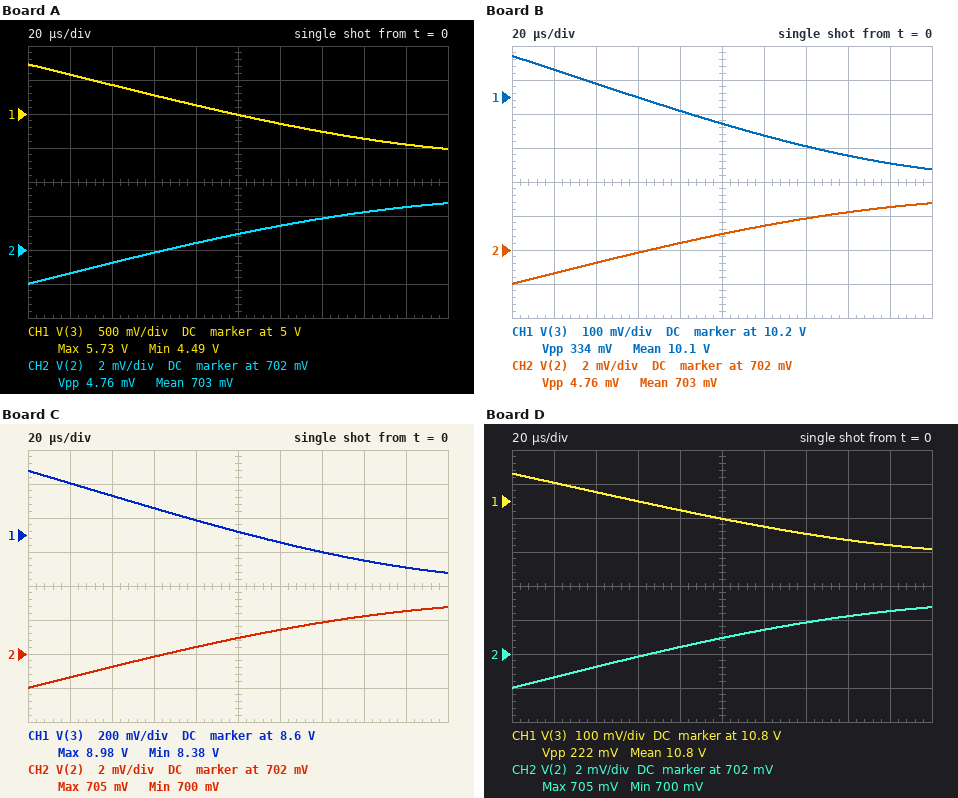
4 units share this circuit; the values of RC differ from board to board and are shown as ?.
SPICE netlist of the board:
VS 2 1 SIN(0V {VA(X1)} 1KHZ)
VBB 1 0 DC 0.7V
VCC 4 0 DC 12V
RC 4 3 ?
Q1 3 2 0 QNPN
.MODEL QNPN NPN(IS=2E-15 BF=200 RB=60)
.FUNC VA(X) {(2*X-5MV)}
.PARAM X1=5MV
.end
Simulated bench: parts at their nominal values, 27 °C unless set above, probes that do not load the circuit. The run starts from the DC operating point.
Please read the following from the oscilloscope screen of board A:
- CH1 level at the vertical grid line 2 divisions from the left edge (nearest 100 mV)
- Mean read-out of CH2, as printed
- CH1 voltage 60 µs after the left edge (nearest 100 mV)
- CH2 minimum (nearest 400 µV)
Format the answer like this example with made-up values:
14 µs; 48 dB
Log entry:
5.4 V; 703 mV; 5.3 V; 700.0 mV
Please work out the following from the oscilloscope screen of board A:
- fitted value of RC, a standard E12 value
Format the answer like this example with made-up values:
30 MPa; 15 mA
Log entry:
5.6 kΩ
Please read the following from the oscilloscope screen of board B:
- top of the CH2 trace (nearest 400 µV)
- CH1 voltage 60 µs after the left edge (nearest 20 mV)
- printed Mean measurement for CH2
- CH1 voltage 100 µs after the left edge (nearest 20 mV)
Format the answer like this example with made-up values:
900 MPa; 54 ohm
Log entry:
704.8 mV; 10.20 V; 703 mV; 10.12 V
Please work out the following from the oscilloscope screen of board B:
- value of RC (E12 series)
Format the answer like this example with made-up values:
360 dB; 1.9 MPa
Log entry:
1.5 kΩ
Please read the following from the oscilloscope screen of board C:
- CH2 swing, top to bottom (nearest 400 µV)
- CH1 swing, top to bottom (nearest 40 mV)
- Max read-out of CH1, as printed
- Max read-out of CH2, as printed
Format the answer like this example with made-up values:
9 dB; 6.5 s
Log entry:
4.8 mV; 600 mV; 8.98 V; 705 mV
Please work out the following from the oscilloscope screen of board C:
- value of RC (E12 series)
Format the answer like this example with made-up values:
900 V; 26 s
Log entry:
2.7 kΩ
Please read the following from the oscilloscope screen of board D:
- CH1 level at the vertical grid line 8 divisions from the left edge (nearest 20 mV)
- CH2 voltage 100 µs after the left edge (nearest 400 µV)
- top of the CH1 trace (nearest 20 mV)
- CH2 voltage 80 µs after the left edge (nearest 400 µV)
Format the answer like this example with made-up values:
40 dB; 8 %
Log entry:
10.68 V; 702.8 mV; 10.88 V; 702.4 mV
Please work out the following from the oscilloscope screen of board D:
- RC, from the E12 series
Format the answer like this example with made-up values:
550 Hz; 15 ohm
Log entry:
1 kΩ
